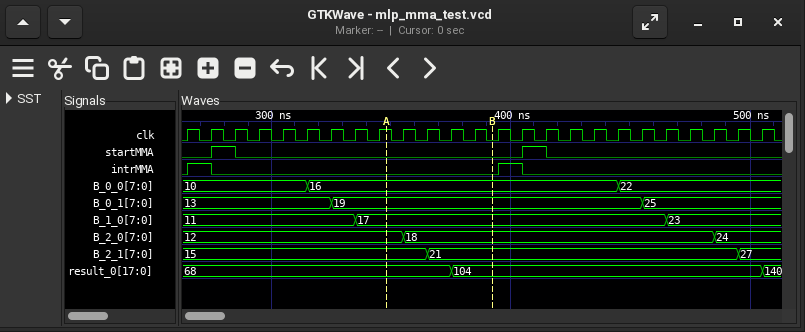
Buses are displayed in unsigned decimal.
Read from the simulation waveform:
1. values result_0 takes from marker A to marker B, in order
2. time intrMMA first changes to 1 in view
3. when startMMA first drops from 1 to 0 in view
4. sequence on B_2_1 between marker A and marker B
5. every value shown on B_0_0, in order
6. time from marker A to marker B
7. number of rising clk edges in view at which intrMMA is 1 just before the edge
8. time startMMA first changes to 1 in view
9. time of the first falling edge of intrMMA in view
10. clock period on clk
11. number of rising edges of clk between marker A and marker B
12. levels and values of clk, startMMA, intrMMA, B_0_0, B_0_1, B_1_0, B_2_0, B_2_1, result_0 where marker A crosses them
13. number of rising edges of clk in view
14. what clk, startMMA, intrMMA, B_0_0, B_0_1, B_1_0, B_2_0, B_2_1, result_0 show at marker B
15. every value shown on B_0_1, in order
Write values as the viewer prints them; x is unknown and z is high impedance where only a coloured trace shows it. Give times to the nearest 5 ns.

68, 104
265 ns
285 ns
15, 21
10, 16, 22
45 ns
2
275 ns
275 ns
10 ns
4
clk=1, startMMA=0, intrMMA=0, B_0_0=16, B_0_1=19, B_1_0=17, B_2_0=12, B_2_1=15, result_0=68
25
clk=0, startMMA=0, intrMMA=0, B_0_0=16, B_0_1=19, B_1_0=17, B_2_0=18, B_2_1=21, result_0=104
13, 19, 25
